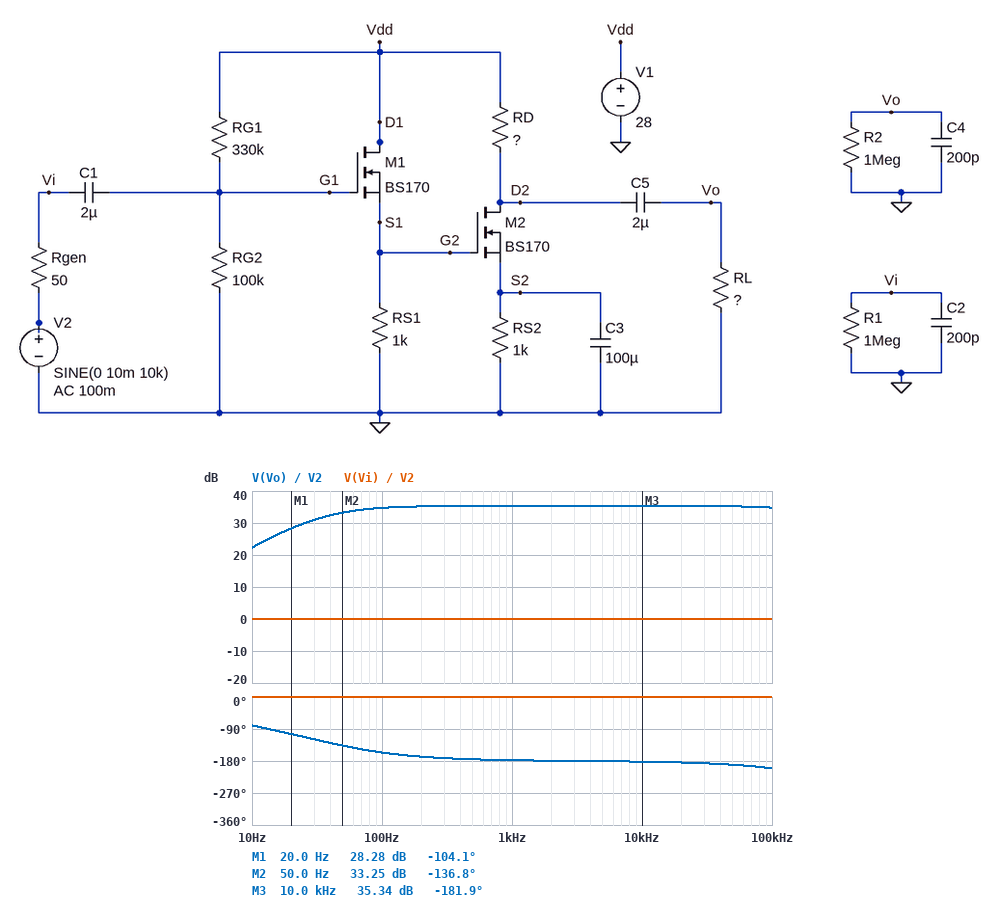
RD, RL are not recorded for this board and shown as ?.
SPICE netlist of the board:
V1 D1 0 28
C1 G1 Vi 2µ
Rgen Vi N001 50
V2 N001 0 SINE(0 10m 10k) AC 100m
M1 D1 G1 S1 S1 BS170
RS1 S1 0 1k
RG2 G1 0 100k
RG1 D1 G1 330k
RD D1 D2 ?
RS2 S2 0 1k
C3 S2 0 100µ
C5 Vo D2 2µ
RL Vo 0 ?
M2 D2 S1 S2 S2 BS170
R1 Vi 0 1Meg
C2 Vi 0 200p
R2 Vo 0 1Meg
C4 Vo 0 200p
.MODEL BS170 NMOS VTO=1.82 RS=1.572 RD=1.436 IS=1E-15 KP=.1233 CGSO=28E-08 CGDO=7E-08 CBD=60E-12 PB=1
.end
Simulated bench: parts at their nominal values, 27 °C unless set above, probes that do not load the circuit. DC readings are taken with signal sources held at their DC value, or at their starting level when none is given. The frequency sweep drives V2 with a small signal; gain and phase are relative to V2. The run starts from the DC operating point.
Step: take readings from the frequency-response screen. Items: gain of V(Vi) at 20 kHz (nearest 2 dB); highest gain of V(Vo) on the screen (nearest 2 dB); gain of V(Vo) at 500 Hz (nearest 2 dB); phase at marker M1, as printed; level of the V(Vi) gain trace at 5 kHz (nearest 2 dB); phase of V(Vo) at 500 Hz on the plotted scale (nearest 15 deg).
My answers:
0 dB
36 dB
36 dB
-104.1 deg
0 dB
-180 deg
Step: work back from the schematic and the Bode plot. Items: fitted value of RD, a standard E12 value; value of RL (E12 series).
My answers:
3.3 kΩ
12 kΩ
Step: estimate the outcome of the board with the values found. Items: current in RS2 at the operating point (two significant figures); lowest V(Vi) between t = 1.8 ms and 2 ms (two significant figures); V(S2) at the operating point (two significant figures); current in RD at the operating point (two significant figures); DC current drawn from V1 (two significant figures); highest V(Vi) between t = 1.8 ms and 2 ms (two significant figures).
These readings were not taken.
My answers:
2.4 mA
-10 mV
2.4 V
2.4 mA
6.9 mA
10 mV
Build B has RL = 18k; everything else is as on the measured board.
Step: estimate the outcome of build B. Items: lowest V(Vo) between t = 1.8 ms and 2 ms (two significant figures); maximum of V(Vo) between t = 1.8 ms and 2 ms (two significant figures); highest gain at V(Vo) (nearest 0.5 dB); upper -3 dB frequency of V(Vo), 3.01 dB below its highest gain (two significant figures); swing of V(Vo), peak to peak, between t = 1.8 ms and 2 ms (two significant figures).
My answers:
-640 mV
620 mV
36.0 dB
250 kHz
1.3 V
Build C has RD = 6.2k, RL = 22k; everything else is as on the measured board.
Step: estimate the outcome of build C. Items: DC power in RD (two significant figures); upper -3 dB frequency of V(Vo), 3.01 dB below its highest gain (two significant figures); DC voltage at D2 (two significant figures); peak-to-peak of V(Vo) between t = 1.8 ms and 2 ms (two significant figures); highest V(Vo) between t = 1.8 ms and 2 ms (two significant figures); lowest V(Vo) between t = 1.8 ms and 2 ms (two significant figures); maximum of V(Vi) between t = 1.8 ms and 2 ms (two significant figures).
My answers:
36 mW
140 kHz
13 V
2.2 V
1.1 V
-1.1 V
10 mV
